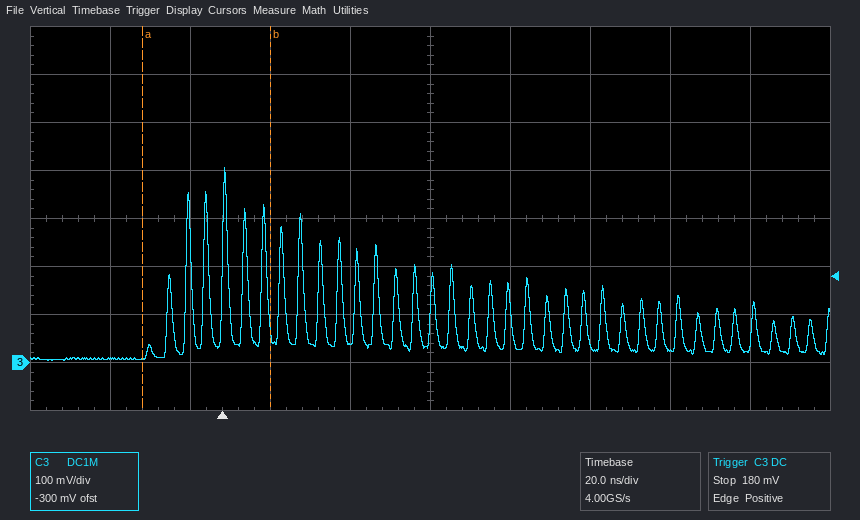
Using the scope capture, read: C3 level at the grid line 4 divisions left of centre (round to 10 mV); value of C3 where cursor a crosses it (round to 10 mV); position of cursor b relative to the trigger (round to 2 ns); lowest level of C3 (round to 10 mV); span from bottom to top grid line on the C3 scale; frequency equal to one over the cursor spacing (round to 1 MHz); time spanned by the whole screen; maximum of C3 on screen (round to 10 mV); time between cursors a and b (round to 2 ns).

10 mV
10 mV
+12 ns
0 mV
800 mV
31 MHz
200 ns
410 mV
32 ns
